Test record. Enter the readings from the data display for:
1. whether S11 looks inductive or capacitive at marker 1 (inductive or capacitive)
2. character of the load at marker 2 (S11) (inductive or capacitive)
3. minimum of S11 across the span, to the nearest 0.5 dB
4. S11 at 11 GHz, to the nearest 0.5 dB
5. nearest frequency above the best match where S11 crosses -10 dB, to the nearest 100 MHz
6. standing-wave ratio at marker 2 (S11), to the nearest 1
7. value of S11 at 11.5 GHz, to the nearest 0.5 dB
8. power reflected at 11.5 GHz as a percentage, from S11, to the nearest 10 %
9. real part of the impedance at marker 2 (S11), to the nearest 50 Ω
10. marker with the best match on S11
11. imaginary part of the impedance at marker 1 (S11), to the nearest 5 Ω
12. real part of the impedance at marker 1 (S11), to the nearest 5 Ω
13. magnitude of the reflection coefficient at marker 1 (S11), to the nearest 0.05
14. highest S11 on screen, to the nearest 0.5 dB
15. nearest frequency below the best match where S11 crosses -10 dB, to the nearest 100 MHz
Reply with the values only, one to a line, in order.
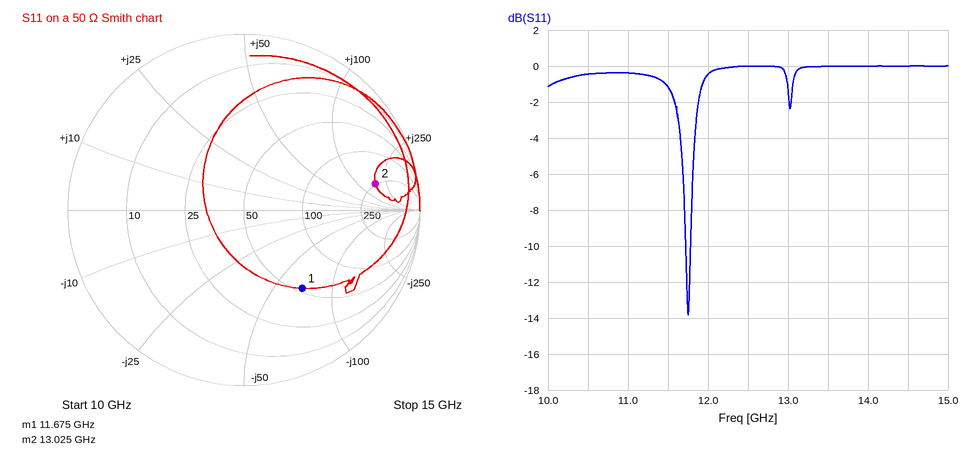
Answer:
capacitive
inductive
-14.0 dB
-0.5 dB
11.8 GHz
7
-1.0 dB
80 %
250 Ω
marker 1
-70 Ω
55 Ω
0.55
0.0 dB
11.7 GHz
